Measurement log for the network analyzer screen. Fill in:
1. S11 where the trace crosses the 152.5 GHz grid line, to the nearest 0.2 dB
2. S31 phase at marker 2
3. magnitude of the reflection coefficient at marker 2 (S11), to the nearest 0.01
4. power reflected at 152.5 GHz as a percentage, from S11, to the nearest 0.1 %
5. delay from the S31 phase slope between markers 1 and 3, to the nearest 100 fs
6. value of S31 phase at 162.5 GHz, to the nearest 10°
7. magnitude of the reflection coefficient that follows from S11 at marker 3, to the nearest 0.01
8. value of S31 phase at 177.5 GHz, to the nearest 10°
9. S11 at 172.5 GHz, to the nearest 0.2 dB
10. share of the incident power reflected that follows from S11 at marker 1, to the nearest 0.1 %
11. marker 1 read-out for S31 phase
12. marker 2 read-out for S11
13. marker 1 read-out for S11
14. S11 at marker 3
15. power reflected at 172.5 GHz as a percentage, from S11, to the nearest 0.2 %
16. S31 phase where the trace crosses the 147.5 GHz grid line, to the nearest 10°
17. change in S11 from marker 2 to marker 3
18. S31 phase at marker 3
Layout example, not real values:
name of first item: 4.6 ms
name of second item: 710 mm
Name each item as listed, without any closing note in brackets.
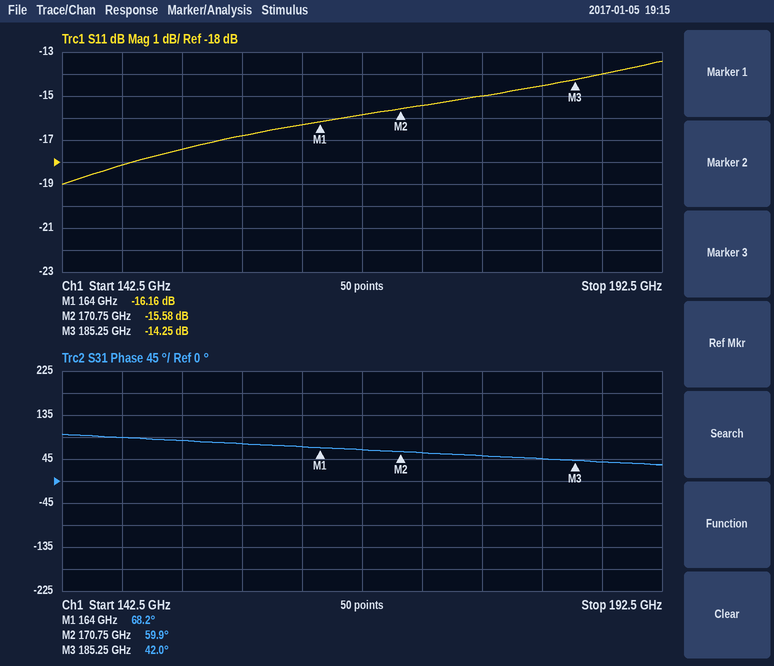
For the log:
S11 where the trace crosses the 152.5 GHz grid line, to the nearest 0.2 dB: -17.4 dB
S31 phase at marker 2: 59.9°
magnitude of the reflection coefficient at marker 2 (S11), to the nearest 0.01: 0.17
power reflected at 152.5 GHz as a percentage, from S11, to the nearest 0.1 %: 1.8 %
delay from the S31 phase slope between markers 1 and 3, to the nearest 100 fs: 3.4 ps
value of S31 phase at 162.5 GHz, to the nearest 10°: 70°
magnitude of the reflection coefficient that follows from S11 at marker 3, to the nearest 0.01: 0.19
value of S31 phase at 177.5 GHz, to the nearest 10°: 50°
S11 at 172.5 GHz, to the nearest 0.2 dB: -15.4 dB
share of the incident power reflected that follows from S11 at marker 1, to the nearest 0.1 %: 2.4 %
marker 1 read-out for S31 phase: 68.2°
marker 2 read-out for S11: -15.58 dB
marker 1 read-out for S11: -16.16 dB
S11 at marker 3: -14.25 dB
power reflected at 172.5 GHz as a percentage, from S11, to the nearest 0.2 %: 2.8 %
S31 phase where the trace crosses the 147.5 GHz grid line, to the nearest 10°: 90°
change in S11 from marker 2 to marker 3: 1.33 dB
S31 phase at marker 3: 42.0°
